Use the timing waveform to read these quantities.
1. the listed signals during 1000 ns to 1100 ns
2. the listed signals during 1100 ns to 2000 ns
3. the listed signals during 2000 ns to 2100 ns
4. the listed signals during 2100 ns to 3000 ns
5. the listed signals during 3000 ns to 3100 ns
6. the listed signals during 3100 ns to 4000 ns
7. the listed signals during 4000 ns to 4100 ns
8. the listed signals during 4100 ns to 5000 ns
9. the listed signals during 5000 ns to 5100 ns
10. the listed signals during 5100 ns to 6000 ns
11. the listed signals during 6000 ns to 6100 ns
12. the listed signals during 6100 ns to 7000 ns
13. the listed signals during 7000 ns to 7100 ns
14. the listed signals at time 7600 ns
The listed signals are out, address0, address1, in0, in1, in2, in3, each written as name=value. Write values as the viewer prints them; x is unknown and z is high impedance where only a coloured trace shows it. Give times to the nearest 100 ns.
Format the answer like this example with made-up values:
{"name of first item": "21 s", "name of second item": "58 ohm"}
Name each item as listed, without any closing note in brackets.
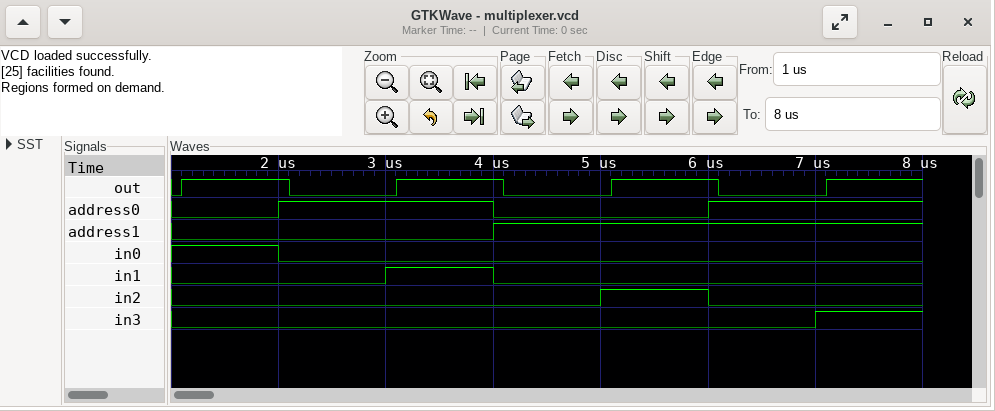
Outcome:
{"the listed signals during 1000 ns to 1100 ns": "out=0, address0=0, address1=0, in0=1, in1=0, in2=0, in3=0", "the listed signals during 1100 ns to 2000 ns": "out=1, address0=0, address1=0, in0=1, in1=0, in2=0, in3=0", "the listed signals during 2000 ns to 2100 ns": "out=1, address0=1, address1=0, in0=0, in1=0, in2=0, in3=0", "the listed signals during 2100 ns to 3000 ns": "out=0, address0=1, address1=0, in0=0, in1=0, in2=0, in3=0", "the listed signals during 3000 ns to 3100 ns": "out=0, address0=1, address1=0, in0=0, in1=1, in2=0, in3=0", "the listed signals during 3100 ns to 4000 ns": "out=1, address0=1, address1=0, in0=0, in1=1, in2=0, in3=0", "the listed signals during 4000 ns to 4100 ns": "out=1, address0=0, address1=1, in0=0, in1=0, in2=0, in3=0", "the listed signals during 4100 ns to 5000 ns": "out=0, address0=0, address1=1, in0=0, in1=0, in2=0, in3=0", "the listed signals during 5000 ns to 5100 ns": "out=0, address0=0, address1=1, in0=0, in1=0, in2=1, in3=0", "the listed signals during 5100 ns to 6000 ns": "out=1, address0=0, address1=1, in0=0, in1=0, in2=1, in3=0", "the listed signals during 6000 ns to 6100 ns": "out=1, address0=1, address1=1, in0=0, in1=0, in2=0, in3=0", "the listed signals during 6100 ns to 7000 ns": "out=0, address0=1, address1=1, in0=0, in1=0, in2=0, in3=0", "the listed signals during 7000 ns to 7100 ns": "out=0, address0=1, address1=1, in0=0, in1=0, in2=0, in3=1", "the listed signals at time 7600 ns": "out=1, address0=1, address1=1, in0=0, in1=0, in2=0, in3=1"}
